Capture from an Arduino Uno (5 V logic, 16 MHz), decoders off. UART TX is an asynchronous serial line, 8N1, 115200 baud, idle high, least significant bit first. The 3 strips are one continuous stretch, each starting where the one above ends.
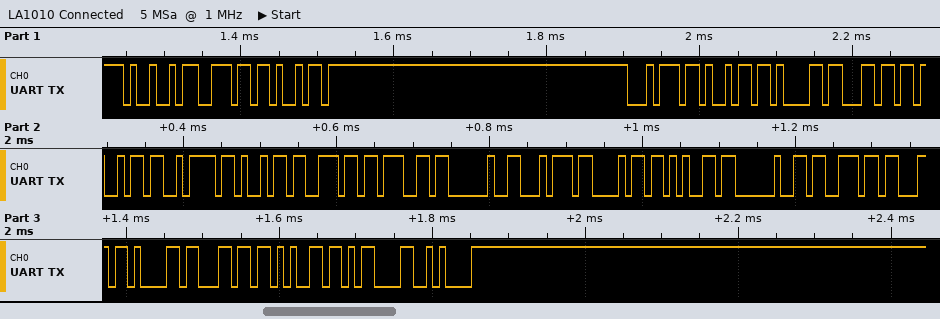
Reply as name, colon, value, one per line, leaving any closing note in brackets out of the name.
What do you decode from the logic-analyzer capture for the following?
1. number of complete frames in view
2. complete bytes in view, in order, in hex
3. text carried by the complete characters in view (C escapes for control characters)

number of complete frames in view: 24
complete bytes in view, in order, in hex: 0x49 0x6E 0x69 0x74 0x69 0x61 0x6C 0x69 0x7A 0x69 0x6E 0x67 0x20 0x74 0x68 0x65 0x20 0x73 0x63 0x61 0x6C 0x65 0x0D 0x0A
text carried by the complete characters in view: "Initializing the scale\r\n"
